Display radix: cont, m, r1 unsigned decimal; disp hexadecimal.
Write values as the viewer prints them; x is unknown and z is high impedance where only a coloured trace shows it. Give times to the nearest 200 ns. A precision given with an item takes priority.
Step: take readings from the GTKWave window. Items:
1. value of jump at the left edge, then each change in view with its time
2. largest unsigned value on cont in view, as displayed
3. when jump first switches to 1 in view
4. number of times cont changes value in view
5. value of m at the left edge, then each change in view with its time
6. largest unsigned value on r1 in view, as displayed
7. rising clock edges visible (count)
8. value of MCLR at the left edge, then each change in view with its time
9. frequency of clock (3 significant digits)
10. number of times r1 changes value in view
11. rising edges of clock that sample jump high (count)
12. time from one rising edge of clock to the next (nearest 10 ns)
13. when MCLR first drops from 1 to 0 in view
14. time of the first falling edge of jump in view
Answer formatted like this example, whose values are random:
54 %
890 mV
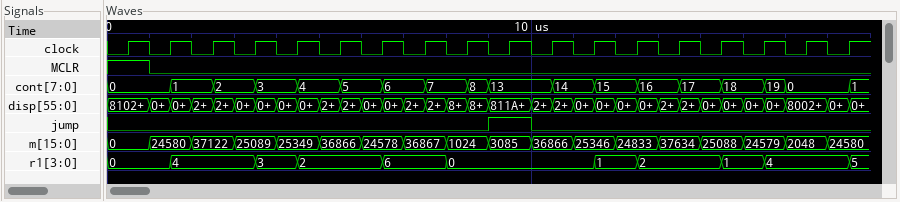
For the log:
0, 1 at 9000 ns, 0 at 10000 ns
19
9000 ns
17
0, 24580 at 1000 ns, 37122 at 2000 ns, 25089 at 3000 ns, 25349 at 4000 ns, 36866 at 5000 ns, 24578 at 6000 ns, 36867 at 7000 ns, 1024 at 8000 ns, 3085 at 9000 ns, 36866 at 10000 ns, 25346 at 11000 ns, 24833 at 12000 ns, 37634 at 13000 ns, 25088 at 14000 ns, 24579 at 15000 ns, 2048 at 16000 ns, 24580 at 17000 ns
6
18
1, 0 at 1000 ns
1.00 MHz
10
1
1000 ns
1000 ns
10000 ns
